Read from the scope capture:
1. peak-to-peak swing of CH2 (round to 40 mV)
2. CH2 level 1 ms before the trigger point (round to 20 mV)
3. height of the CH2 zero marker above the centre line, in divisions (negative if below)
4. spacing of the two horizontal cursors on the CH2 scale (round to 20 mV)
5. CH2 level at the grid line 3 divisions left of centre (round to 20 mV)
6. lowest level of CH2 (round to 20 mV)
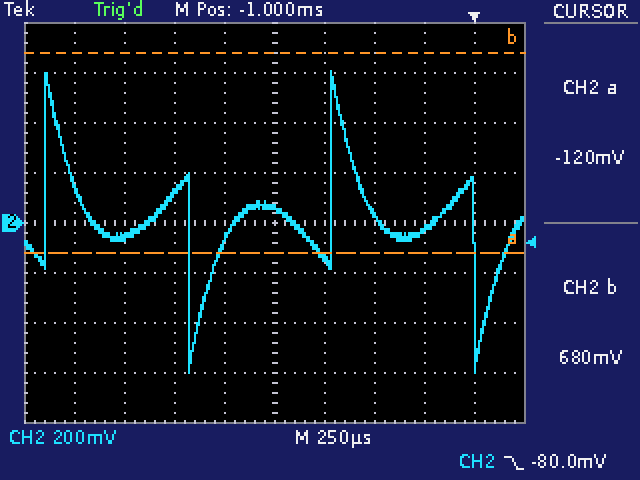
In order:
1.20 V
60 mV
0.0 div
800 mV
-60 mV
-600 mV
